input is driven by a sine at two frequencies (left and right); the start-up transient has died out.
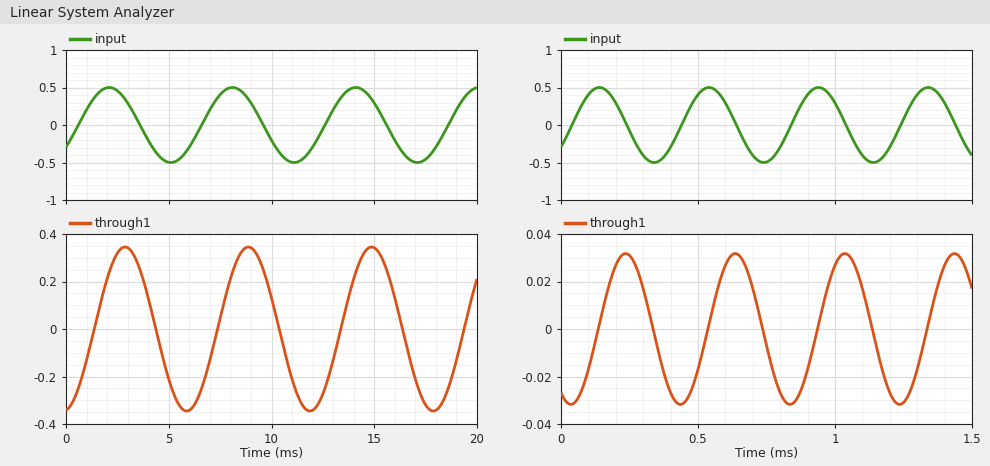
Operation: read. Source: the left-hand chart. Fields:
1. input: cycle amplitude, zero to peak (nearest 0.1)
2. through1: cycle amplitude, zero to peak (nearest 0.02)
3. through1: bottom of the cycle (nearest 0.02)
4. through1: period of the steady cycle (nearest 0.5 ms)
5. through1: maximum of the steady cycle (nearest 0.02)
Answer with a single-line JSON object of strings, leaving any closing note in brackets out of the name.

{"input: cycle amplitude, zero to peak": "0.5", "through1: cycle amplitude, zero to peak": "0.34", "through1: bottom of the cycle": "-0.34", "through1: period of the steady cycle": "6.0 ms", "through1: maximum of the steady cycle": "0.34"}
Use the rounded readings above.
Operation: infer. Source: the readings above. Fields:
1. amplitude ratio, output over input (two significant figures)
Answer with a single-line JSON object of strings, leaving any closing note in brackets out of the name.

{"amplitude ratio, output over input": "0.68"}
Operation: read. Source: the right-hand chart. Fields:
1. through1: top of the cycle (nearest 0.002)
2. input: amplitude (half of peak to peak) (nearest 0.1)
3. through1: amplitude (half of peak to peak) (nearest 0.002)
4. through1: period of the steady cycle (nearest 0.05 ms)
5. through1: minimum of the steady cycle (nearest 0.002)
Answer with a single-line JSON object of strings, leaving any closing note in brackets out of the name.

{"through1: top of the cycle": "0.032", "input: amplitude (half of peak to peak)": "0.5", "through1: amplitude (half of peak to peak)": "0.032", "through1: period of the steady cycle": "0.40 ms", "through1: minimum of the steady cycle": "-0.032"}
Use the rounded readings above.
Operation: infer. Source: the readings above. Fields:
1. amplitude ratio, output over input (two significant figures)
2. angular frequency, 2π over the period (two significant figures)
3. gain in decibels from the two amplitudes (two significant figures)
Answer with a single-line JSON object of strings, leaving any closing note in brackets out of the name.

{"amplitude ratio, output over input": "0.064", "angular frequency, 2π over the period": "16 rad/ms", "gain in decibels from the two amplitudes": "-24 dB"}
